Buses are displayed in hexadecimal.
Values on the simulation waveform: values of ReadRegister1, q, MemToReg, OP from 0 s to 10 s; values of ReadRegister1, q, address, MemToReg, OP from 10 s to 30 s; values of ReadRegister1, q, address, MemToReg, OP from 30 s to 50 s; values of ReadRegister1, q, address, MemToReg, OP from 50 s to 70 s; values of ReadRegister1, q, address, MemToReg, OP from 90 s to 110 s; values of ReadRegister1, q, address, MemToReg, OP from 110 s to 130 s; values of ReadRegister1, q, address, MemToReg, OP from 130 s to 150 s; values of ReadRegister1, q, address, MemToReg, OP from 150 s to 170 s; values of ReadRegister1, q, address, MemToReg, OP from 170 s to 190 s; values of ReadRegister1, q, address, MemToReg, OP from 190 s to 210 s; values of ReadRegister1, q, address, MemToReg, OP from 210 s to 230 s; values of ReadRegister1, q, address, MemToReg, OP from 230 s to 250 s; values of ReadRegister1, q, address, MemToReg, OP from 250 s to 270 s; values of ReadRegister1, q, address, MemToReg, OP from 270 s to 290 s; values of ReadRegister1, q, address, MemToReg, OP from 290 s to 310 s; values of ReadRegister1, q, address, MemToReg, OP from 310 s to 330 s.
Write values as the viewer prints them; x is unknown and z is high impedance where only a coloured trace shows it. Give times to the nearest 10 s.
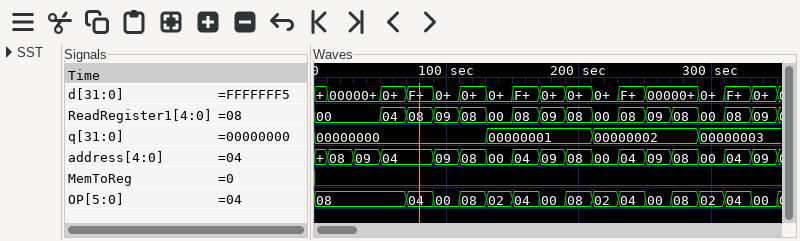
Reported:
ReadRegister1=00, q=00000000, MemToReg=0, OP=08
ReadRegister1=00, q=00000000, address=08, MemToReg=0, OP=08
ReadRegister1=00, q=00000000, address=09, MemToReg=0, OP=08
ReadRegister1=04, q=00000000, address=04, MemToReg=0, OP=08
ReadRegister1=09, q=00000000, address=09, MemToReg=0, OP=00
ReadRegister1=08, q=00000000, address=08, MemToReg=0, OP=08
ReadRegister1=00, q=00000001, address=00, MemToReg=0, OP=02
ReadRegister1=08, q=00000001, address=04, MemToReg=0, OP=04
ReadRegister1=09, q=00000001, address=09, MemToReg=0, OP=00
ReadRegister1=08, q=00000001, address=08, MemToReg=0, OP=08
ReadRegister1=00, q=00000002, address=00, MemToReg=0, OP=02
ReadRegister1=08, q=00000002, address=04, MemToReg=0, OP=04
ReadRegister1=09, q=00000002, address=09, MemToReg=0, OP=00
ReadRegister1=08, q=00000002, address=08, MemToReg=0, OP=08
ReadRegister1=00, q=00000003, address=00, MemToReg=0, OP=02
ReadRegister1=08, q=00000003, address=04, MemToReg=0, OP=04
